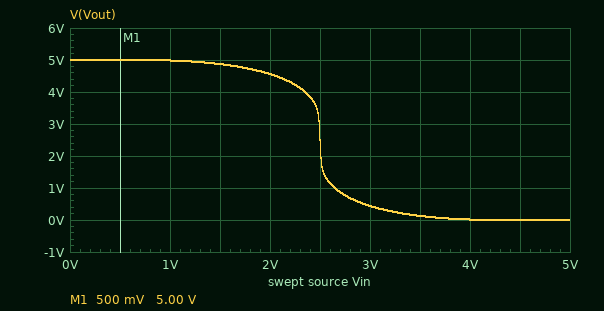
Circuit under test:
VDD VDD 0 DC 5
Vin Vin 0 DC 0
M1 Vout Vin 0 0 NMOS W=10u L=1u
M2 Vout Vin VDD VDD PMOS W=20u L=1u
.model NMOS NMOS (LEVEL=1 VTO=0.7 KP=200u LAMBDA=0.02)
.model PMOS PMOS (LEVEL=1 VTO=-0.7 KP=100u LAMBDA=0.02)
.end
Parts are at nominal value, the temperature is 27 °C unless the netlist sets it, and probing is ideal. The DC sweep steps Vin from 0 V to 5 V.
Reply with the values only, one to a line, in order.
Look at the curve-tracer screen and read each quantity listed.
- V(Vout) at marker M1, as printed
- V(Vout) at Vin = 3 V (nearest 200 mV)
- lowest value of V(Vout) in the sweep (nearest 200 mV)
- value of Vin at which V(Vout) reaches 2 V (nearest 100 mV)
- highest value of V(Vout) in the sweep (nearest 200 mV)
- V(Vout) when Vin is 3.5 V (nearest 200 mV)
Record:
5.00 V
400 mV
0 V
2.5 V
5.0 V
200 mV
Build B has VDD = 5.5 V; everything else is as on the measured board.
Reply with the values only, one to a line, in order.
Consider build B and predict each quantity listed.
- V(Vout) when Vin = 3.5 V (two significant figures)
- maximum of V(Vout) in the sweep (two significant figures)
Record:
350 mV
5.5 V
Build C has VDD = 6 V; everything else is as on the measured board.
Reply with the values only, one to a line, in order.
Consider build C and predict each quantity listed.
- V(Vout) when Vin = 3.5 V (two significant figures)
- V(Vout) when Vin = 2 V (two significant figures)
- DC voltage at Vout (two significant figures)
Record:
720 mV
5.7 V
6.0 V
